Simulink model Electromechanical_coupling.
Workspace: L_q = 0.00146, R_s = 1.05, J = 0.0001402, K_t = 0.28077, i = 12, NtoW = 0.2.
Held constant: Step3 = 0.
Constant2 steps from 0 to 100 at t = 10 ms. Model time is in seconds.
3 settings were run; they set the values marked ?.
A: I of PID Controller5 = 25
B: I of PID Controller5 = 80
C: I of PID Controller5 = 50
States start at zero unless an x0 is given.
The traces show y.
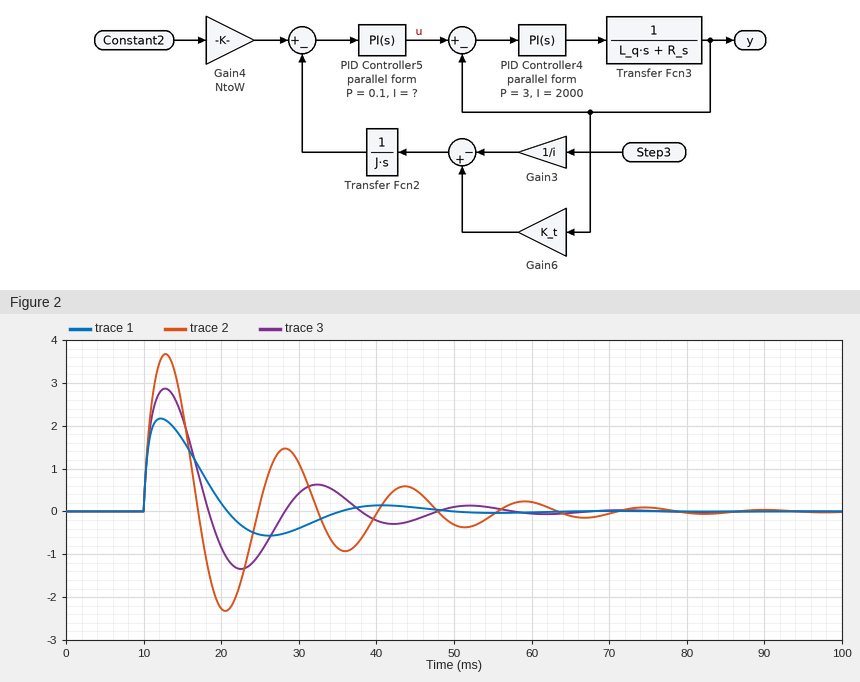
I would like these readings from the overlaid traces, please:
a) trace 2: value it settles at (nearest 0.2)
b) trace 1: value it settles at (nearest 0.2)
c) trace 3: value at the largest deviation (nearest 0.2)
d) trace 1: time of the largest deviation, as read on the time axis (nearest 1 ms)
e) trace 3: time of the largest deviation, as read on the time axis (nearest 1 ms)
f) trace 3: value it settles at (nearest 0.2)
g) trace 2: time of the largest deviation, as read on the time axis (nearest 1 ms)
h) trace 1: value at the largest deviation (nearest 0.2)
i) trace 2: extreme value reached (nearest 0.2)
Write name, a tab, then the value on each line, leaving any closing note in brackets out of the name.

trace 2: value it settles at	0.0
trace 1: value it settles at	0.0
trace 3: value at the largest deviation	2.8
trace 1: time of the largest deviation, as read on the time axis	12 ms
trace 3: time of the largest deviation, as read on the time axis	13 ms
trace 3: value it settles at	0.0
trace 2: time of the largest deviation, as read on the time axis	13 ms
trace 1: value at the largest deviation	2.2
trace 2: extreme value reached	3.6
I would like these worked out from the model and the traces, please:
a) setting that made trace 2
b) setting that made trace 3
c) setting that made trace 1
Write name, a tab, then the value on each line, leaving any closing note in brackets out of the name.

setting that made trace 2	B
setting that made trace 3	C
setting that made trace 1	A
